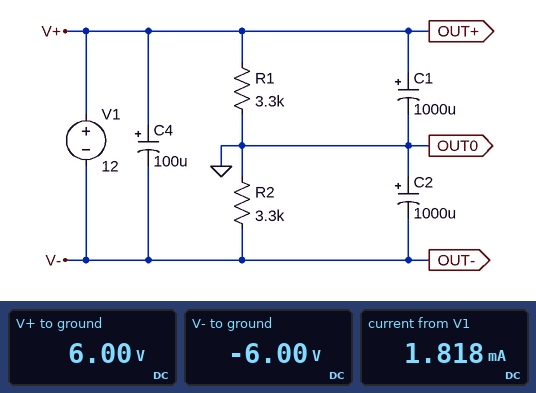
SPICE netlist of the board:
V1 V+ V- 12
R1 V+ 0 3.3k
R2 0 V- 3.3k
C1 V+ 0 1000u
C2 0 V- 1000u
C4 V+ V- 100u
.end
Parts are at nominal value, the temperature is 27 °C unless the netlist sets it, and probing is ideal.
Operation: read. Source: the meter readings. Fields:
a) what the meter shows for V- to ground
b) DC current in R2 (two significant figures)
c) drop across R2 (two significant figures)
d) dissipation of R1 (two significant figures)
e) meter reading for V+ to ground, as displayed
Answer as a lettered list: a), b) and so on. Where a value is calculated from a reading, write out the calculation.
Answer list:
a) -6.00 V
b) (0 V - (-6 V)) / 3.3 kΩ = 1.8 mA
c) 0 V - (-6 V) = 6.0 V
d) (6 V)^2 / 3.3 kΩ = 11 mW
e) 6.00 V
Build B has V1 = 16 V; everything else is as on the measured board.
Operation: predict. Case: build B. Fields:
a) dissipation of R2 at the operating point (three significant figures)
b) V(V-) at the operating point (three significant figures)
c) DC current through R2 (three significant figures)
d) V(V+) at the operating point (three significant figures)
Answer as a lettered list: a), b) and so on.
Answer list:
a) 19.4 mW
b) -8.00 V
c) 2.42 mA
d) 8.00 V
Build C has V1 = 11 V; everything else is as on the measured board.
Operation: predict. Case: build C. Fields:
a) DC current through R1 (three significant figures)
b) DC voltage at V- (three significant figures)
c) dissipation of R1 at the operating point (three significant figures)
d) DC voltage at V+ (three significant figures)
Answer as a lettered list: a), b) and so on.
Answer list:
a) 1.67 mA
b) -5.50 V
c) 9.17 mW
d) 5.50 V
